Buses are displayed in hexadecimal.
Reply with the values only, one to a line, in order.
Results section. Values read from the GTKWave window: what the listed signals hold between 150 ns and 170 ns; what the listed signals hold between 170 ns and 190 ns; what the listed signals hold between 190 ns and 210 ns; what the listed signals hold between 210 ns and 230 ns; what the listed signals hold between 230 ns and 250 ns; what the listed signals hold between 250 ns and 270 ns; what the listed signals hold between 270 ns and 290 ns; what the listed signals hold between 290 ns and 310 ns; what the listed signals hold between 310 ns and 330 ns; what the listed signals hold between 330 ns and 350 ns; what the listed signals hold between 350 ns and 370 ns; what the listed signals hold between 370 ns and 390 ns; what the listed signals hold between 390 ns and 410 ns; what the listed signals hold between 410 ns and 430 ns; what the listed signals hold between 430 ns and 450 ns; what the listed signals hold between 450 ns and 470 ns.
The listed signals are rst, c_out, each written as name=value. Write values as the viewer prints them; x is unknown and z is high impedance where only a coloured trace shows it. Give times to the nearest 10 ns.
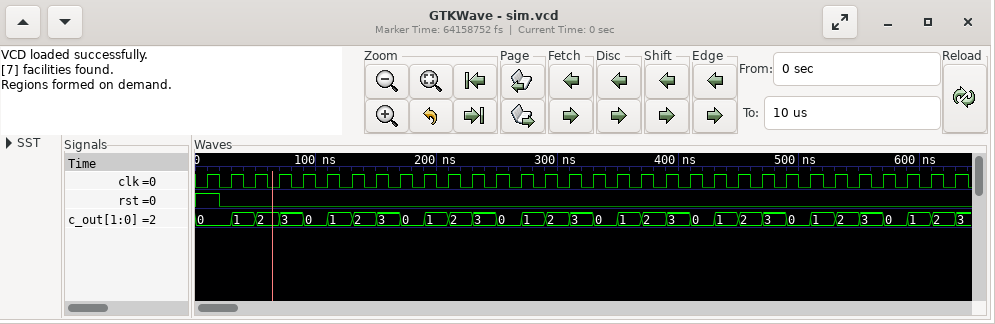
rst=0, c_out=3
rst=0, c_out=0
rst=0, c_out=1
rst=0, c_out=2
rst=0, c_out=3
rst=0, c_out=0
rst=0, c_out=1
rst=0, c_out=2
rst=0, c_out=3
rst=0, c_out=0
rst=0, c_out=1
rst=0, c_out=2
rst=0, c_out=3
rst=0, c_out=0
rst=0, c_out=1
rst=0, c_out=2
